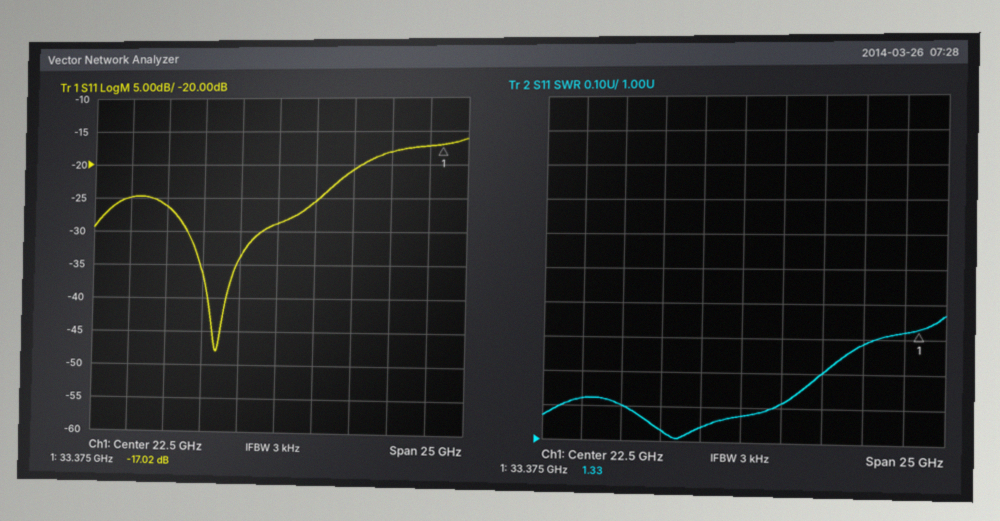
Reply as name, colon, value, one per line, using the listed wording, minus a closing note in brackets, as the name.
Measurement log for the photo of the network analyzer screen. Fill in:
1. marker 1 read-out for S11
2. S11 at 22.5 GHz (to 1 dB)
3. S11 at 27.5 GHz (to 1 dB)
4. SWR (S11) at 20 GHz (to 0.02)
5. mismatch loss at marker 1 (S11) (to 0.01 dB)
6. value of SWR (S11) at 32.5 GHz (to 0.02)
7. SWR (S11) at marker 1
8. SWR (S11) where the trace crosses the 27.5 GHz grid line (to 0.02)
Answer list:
marker 1 read-out for S11: -17.02 dB
S11 at 22.5 GHz: -29 dB
S11 at 27.5 GHz: -21 dB
SWR (S11) at 20 GHz: 1.04
mismatch loss at marker 1 (S11): 0.09 dB
value of SWR (S11) at 32.5 GHz: 1.32
SWR (S11) at marker 1: 1.33
SWR (S11) where the trace crosses the 27.5 GHz grid line: 1.20
